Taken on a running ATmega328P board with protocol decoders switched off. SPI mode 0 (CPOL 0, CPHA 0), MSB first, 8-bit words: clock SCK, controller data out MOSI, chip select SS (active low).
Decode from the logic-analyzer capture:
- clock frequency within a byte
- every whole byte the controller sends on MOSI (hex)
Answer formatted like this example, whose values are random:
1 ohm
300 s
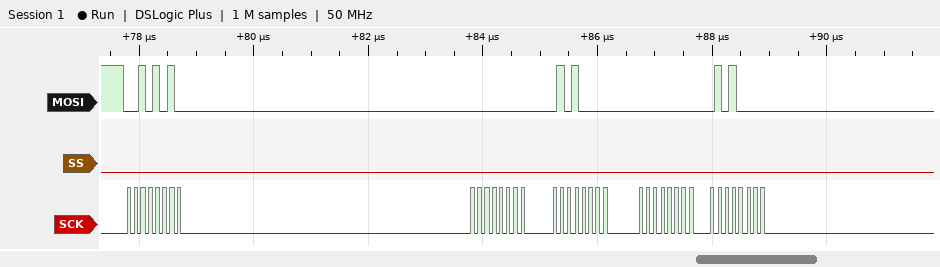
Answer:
8 MHz
2A 00 50 00 50
